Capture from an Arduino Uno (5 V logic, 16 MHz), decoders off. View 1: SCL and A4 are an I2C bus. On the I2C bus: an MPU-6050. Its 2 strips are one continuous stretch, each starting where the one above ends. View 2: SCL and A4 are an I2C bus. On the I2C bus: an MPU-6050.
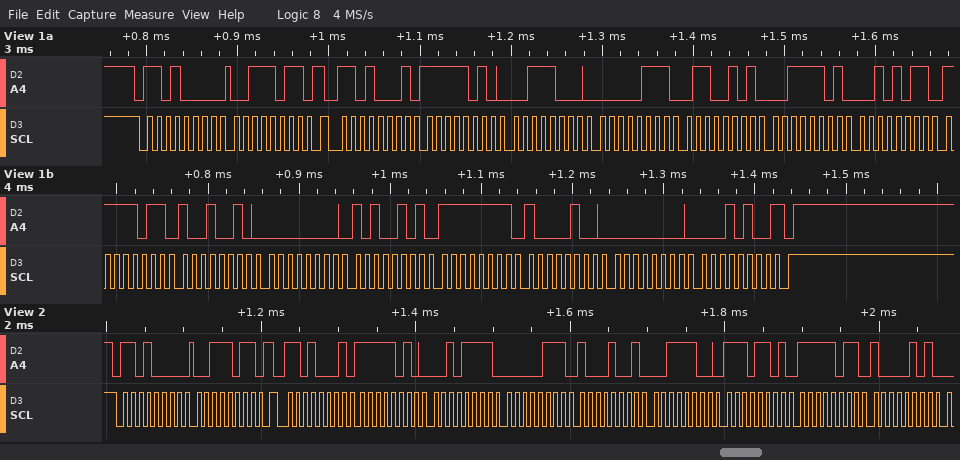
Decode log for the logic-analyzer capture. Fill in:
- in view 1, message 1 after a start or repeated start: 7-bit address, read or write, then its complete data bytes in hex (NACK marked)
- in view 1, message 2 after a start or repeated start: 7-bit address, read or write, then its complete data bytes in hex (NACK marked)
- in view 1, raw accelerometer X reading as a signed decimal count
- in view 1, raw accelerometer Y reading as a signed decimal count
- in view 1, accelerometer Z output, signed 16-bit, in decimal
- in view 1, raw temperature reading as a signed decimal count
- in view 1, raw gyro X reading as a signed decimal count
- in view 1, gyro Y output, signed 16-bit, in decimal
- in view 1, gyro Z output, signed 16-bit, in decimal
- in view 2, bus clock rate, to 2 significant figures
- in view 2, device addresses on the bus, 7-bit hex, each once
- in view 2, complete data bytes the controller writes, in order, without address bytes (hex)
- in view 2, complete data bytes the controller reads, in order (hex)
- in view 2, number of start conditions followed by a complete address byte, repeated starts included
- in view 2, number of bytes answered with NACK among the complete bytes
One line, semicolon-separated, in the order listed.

0x68 write: 3B; 0x68 read: FA 38 07 65 3D 2B FB 92 00 A5 FF 84 00 14 NACK; -1480; 1893; 15659; -1134; 165; -124; 20; 100 kHz; 0x68; 3B; FA 2F 07 89 3C ED FB 85; 2; 0
